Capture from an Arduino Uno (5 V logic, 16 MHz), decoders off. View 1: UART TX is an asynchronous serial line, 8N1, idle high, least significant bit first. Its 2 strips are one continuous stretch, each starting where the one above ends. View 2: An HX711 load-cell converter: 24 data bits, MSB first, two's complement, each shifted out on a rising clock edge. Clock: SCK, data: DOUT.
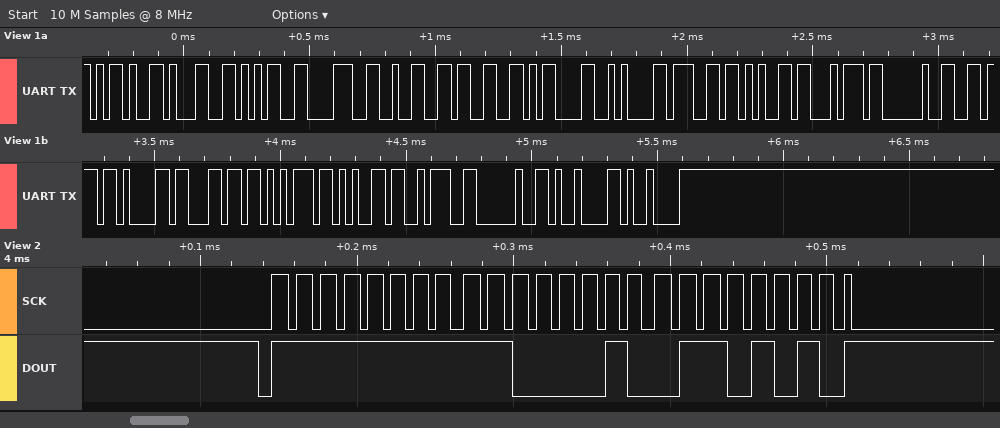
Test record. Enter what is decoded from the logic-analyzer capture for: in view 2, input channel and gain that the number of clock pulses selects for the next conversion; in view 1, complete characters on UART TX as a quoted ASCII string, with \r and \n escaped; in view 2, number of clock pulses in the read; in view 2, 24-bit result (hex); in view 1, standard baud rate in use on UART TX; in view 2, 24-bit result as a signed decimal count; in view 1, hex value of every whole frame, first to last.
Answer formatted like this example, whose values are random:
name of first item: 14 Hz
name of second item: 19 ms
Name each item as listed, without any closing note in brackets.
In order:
in view 2, input channel and gain that the number of clock pulses selects for the next conversion: channel A, gain 128
in view 1, complete characters on UART TX as a quoted ASCII string, with \r and \n escaped: "-15823\r\nget value: \t\t"
in view 2, number of clock pulses in the read: 25
in view 2, 24-bit result: 0xFFC26A
in view 1, standard baud rate in use on UART TX: 38400 baud
in view 2, 24-bit result as a signed decimal count: -15766
in view 1, hex value of every whole frame, first to last: 2D 31 35 38 32 33 0D 0A 67 65 74 20 76 61 6C 75 65 3A 20 09 09
